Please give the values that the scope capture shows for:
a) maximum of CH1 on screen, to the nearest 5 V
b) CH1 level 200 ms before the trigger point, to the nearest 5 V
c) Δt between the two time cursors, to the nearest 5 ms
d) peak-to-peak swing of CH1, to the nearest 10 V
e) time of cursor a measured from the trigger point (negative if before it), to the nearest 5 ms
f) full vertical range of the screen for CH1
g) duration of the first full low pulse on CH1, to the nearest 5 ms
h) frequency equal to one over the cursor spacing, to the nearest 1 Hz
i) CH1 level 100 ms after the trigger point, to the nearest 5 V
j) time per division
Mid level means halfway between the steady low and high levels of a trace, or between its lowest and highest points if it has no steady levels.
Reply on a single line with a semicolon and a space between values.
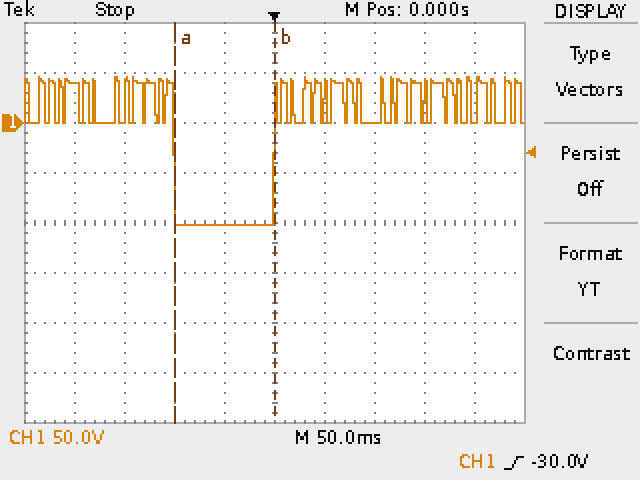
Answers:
45 V; 40 V; 100 ms; 150 V; -100 ms; 400 V; 100 ms; 10 Hz; 0 V; 50 ms
